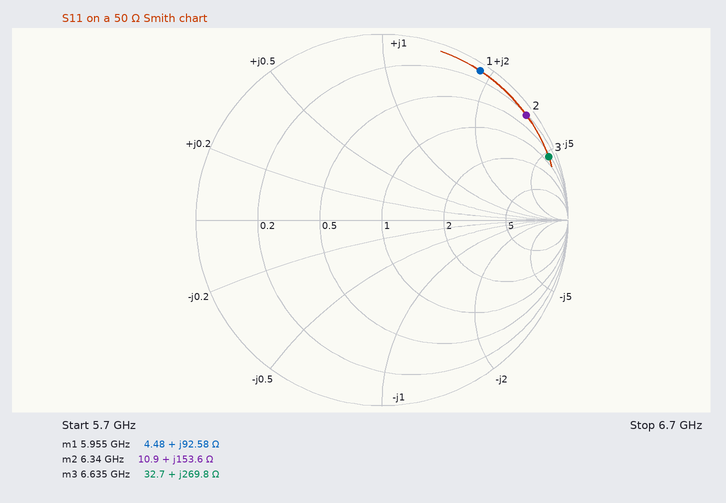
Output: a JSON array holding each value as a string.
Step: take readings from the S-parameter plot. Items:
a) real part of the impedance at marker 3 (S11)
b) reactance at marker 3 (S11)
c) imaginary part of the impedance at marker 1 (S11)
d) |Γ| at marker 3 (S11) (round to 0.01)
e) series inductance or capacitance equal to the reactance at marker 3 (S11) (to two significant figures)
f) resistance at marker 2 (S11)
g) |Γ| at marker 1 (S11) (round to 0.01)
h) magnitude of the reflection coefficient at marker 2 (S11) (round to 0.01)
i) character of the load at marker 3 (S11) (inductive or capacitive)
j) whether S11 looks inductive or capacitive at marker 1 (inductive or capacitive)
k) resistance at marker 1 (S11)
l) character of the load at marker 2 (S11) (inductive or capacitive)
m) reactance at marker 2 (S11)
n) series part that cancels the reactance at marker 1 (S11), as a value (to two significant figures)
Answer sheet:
["32.7 Ω", "+269.8 Ω", "+92.58 Ω", "0.96", "6.5 nH", "10.9 Ω", "0.96", "0.96", "inductive", "inductive", "4.48 Ω", "inductive", "+153.6 Ω", "290 fF"]
